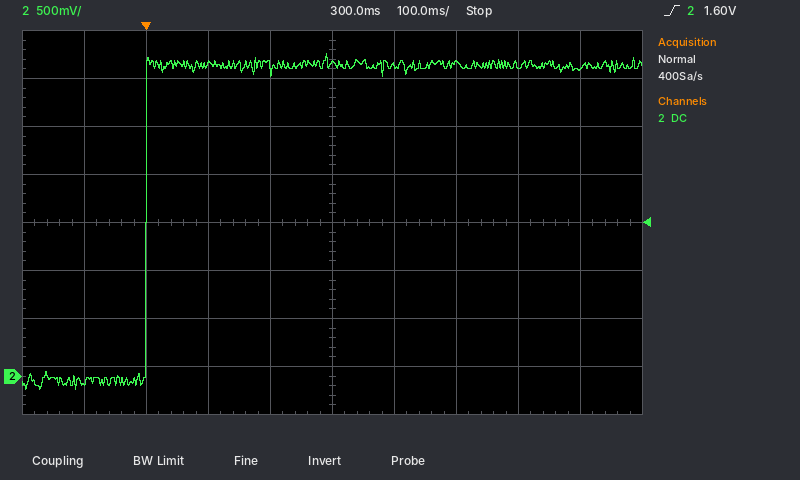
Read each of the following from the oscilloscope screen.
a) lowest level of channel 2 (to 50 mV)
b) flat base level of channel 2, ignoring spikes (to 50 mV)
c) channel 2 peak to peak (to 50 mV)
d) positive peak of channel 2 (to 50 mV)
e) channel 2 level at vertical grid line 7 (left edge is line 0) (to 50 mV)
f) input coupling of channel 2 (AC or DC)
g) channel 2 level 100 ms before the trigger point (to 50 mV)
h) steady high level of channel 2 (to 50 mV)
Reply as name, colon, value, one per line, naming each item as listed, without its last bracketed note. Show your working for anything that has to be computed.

lowest level of channel 2: -150 mV
flat base level of channel 2, ignoring spikes: -50 mV
channel 2 peak to peak: 3.35 V − (-150 mV) = 3.50 V
positive peak of channel 2: 3.35 V
channel 2 level at vertical grid line 7 (left edge is line 0): 3.25 V
input coupling of channel 2: DC
channel 2 level 100 ms before the trigger point: -50 mV
steady high level of channel 2: 3.25 V
